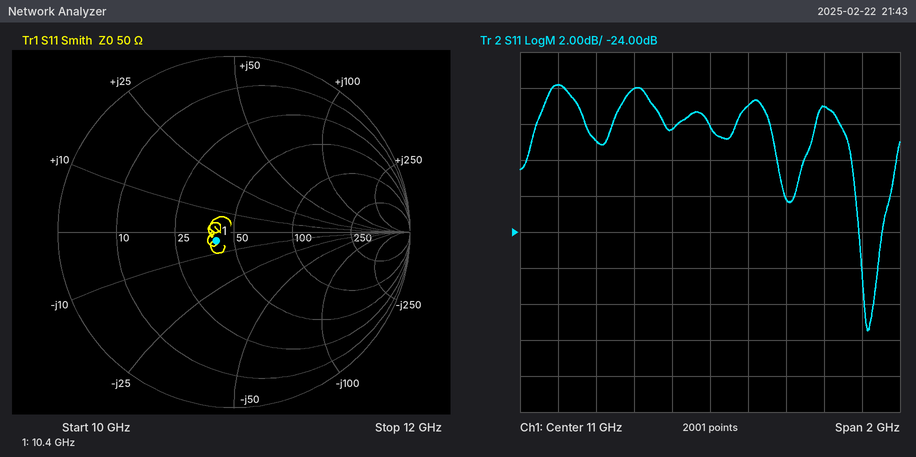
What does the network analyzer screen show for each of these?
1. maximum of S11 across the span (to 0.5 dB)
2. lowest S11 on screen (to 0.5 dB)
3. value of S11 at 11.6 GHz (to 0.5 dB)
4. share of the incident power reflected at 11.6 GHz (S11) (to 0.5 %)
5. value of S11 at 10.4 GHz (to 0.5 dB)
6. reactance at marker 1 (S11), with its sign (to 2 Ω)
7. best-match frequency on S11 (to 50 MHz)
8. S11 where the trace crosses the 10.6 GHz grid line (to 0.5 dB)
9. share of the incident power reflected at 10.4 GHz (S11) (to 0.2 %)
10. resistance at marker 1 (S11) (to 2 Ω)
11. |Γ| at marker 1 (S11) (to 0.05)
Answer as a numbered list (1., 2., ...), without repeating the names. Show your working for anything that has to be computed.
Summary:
1. -16.0 dB
2. -29.5 dB
3. -17.0 dB
4. 10^(-17/10) ≈ 2.0 %
5. -19.0 dB
6. -4 Ω
7. 11.85 GHz
8. -16.0 dB
9. 10^(-19/10) ≈ 1.26 %, so 1.2 % to the nearest 0.2 %
10. 40 Ω
11. 0.10
